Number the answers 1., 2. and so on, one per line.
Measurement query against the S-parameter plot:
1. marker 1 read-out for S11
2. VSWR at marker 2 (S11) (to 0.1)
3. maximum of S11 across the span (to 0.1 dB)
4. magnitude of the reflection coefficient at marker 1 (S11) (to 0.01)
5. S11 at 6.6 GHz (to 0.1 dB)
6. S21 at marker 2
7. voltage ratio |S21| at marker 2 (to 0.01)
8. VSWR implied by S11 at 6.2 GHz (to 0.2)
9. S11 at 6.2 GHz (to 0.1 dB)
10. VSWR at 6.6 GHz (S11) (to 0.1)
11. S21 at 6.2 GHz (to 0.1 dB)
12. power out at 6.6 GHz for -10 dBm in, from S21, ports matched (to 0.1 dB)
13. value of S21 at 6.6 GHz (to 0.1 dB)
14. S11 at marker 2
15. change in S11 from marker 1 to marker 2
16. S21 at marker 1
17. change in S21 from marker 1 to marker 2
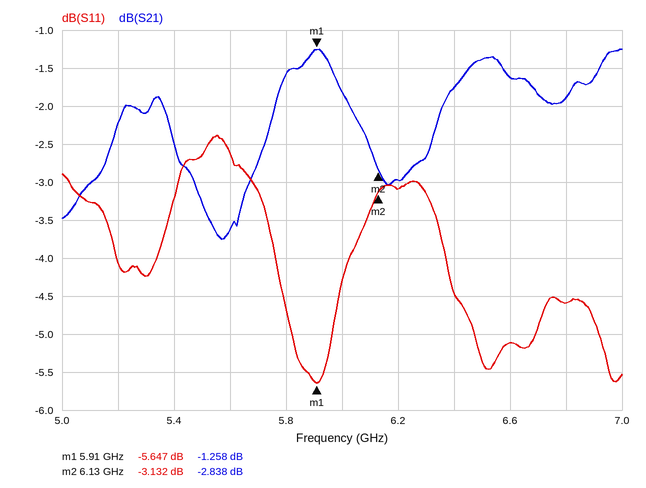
1. -5.647 dB
2. 5.6
3. -2.4 dB
4. 0.52
5. -5.1 dB
6. -2.838 dB
7. 0.72
8. 5.6
9. -3.1 dB
10. 3.5
11. -3.0 dB
12. -11.6 dBm
13. -1.6 dB
14. -3.132 dB
15. 2.515 dB
16. -1.258 dB
17. -1.580 dB
